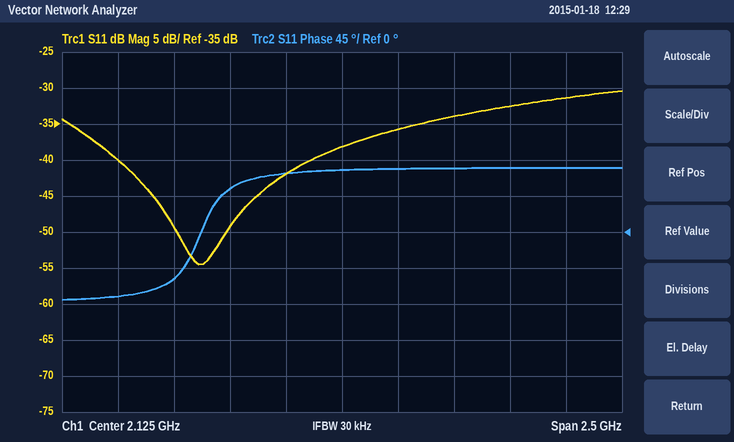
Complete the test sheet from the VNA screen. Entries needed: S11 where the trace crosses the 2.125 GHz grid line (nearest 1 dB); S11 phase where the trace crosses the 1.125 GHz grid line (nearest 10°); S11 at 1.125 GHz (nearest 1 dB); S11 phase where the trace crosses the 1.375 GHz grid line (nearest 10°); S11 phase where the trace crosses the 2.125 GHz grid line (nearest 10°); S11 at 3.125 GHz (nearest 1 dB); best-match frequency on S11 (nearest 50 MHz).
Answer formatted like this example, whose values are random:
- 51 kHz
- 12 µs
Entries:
- -38 dB
- -80°
- -40 dB
- -60°
- 80°
- -31 dB
- 1.50 GHz
